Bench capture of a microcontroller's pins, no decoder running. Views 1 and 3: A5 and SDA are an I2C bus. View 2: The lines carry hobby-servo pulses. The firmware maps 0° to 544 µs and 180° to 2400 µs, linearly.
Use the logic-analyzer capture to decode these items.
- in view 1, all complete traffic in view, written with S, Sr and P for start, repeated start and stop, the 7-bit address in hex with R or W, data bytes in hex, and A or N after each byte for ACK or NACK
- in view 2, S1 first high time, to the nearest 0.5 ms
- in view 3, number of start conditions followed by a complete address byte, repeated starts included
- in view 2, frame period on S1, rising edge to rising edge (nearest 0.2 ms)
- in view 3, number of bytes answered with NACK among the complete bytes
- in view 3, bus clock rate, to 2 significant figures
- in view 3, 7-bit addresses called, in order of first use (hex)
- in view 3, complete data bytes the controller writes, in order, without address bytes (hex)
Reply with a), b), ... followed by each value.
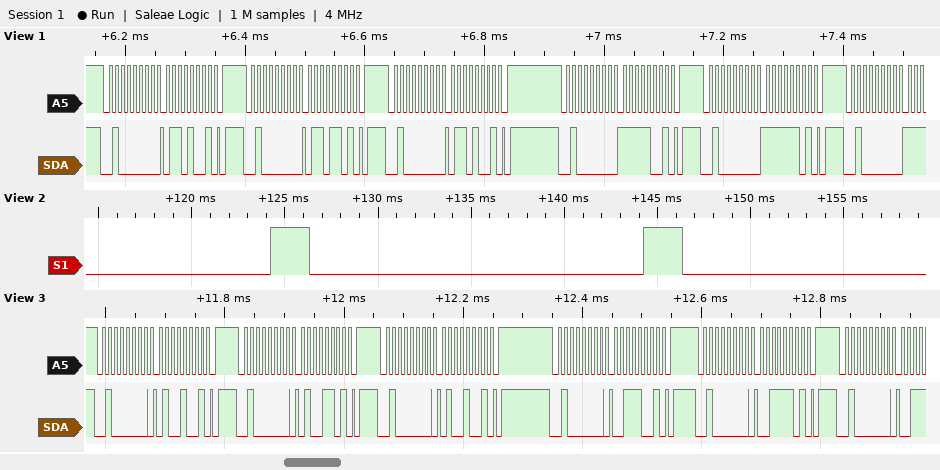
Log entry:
a) S 20W A 69 A P S 20W A 6D A P S 20W A 69 A P S 20W A F9 A P S 20W A FD A P S 20W A
b) 2.0 ms
c) 6
d) 20.0 ms
e) 0
f) 100 kHz
g) 0x20
h) 49 4D 49 39 3D
